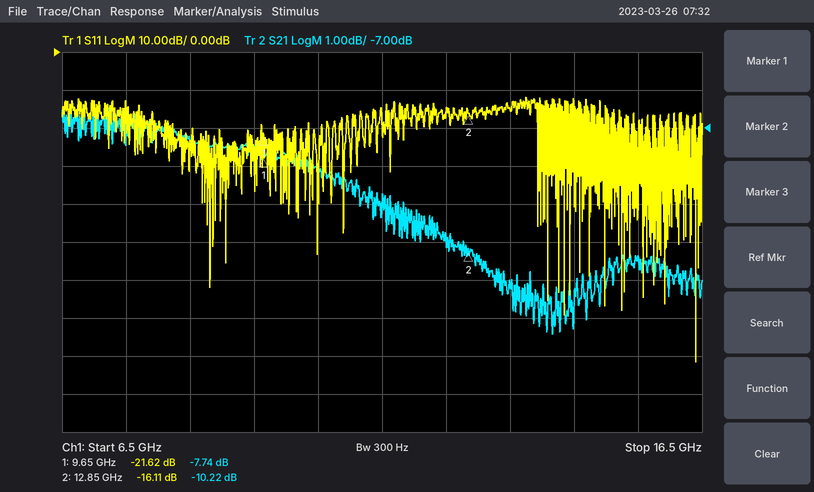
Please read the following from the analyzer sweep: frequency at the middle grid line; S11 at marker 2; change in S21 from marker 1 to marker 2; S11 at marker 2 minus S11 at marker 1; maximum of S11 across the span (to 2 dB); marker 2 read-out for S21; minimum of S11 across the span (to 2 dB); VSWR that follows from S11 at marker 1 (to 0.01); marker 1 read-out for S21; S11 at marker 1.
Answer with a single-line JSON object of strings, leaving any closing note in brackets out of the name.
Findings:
{"frequency at the middle grid line": "11.5 GHz", "S11 at marker 2": "-16.11 dB", "change in S21 from marker 1 to marker 2": "-2.48 dB", "S11 at marker 2 minus S11 at marker 1": "5.51 dB", "maximum of S11 across the span": "-12 dB", "marker 2 read-out for S21": "-10.22 dB", "minimum of S11 across the span": "-82 dB", "VSWR that follows from S11 at marker 1": "1.18", "marker 1 read-out for S21": "-7.74 dB", "S11 at marker 1": "-21.62 dB"}
